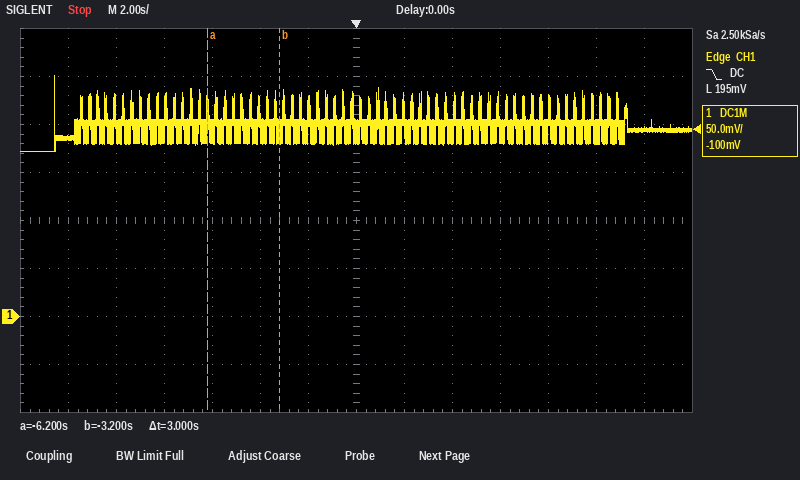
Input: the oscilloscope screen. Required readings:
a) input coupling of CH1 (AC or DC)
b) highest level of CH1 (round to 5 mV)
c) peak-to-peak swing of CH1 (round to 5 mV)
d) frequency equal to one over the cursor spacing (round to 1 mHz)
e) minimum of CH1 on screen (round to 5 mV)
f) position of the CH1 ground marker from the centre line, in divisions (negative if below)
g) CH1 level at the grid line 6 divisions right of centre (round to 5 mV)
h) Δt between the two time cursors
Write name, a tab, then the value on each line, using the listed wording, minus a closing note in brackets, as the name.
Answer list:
input coupling of CH1	DC
highest level of CH1	250 mV
peak-to-peak swing of CH1	80 mV
frequency equal to one over the cursor spacing	333 mHz
minimum of CH1 on screen	170 mV
position of the CH1 ground marker from the centre line, in divisions	-2.0 div
CH1 level at the grid line 6 divisions right of centre	195 mV
Δt between the two time cursors	3 s
